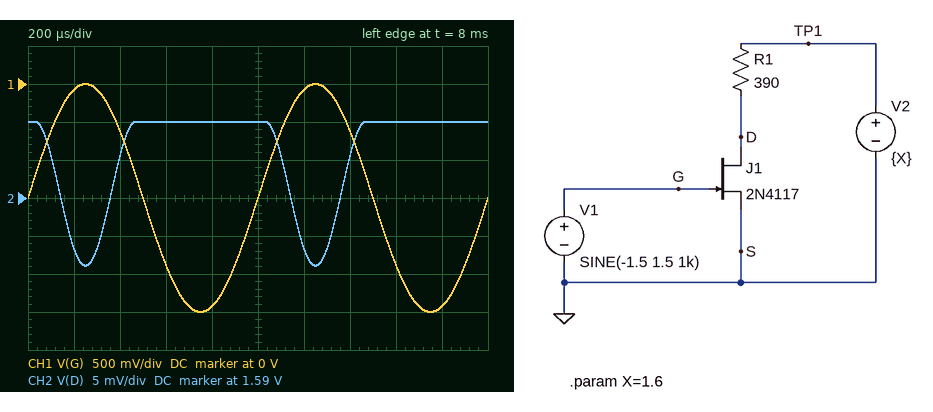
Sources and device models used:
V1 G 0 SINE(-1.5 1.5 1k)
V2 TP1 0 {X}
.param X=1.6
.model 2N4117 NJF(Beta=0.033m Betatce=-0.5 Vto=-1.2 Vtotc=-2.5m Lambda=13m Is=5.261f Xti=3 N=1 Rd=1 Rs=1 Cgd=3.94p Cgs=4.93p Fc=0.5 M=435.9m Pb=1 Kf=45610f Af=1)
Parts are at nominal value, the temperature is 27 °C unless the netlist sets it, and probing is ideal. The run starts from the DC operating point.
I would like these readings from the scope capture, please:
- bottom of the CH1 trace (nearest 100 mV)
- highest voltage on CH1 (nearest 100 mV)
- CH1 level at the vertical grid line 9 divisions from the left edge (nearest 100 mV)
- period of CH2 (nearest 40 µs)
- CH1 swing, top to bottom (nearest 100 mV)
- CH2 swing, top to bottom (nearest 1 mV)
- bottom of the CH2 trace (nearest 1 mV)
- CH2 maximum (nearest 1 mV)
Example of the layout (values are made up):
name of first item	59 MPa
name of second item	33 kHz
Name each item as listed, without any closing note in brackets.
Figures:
bottom of the CH1 trace	-3.0 V
highest voltage on CH1	0 V
CH1 level at the vertical grid line 9 divisions from the left edge	-2.9 V
period of CH2	1.00 ms
CH1 swing, top to bottom	3.0 V
CH2 swing, top to bottom	19 mV
bottom of the CH2 trace	1.581 V
CH2 maximum	1.600 V
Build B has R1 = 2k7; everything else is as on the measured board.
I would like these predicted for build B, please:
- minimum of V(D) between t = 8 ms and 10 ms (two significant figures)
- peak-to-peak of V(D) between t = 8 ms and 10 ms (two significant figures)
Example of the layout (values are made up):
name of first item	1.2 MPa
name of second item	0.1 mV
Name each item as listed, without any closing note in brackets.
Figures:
minimum of V(D) between t = 8 ms and 10 ms	1.5 V
peak-to-peak of V(D) between t = 8 ms and 10 ms	130 mV
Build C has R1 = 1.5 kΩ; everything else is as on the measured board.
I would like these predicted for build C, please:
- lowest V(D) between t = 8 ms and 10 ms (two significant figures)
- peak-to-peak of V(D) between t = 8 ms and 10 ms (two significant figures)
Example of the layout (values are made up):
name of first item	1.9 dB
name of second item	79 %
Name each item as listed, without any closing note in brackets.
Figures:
lowest V(D) between t = 8 ms and 10 ms	1.5 V
peak-to-peak of V(D) between t = 8 ms and 10 ms	73 mV
